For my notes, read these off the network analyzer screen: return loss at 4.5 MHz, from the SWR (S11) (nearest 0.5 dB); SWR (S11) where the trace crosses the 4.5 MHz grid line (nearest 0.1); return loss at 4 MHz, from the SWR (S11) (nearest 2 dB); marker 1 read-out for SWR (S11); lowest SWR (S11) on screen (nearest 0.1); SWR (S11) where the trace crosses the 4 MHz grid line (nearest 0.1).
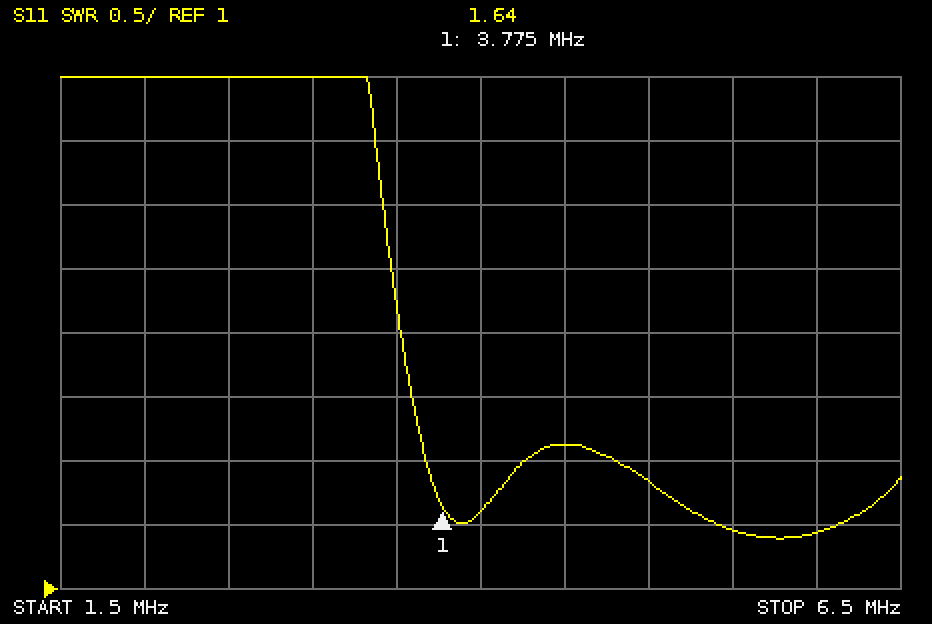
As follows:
9.0 dB
2.1
12 dB
1.64
1.4
1.6
